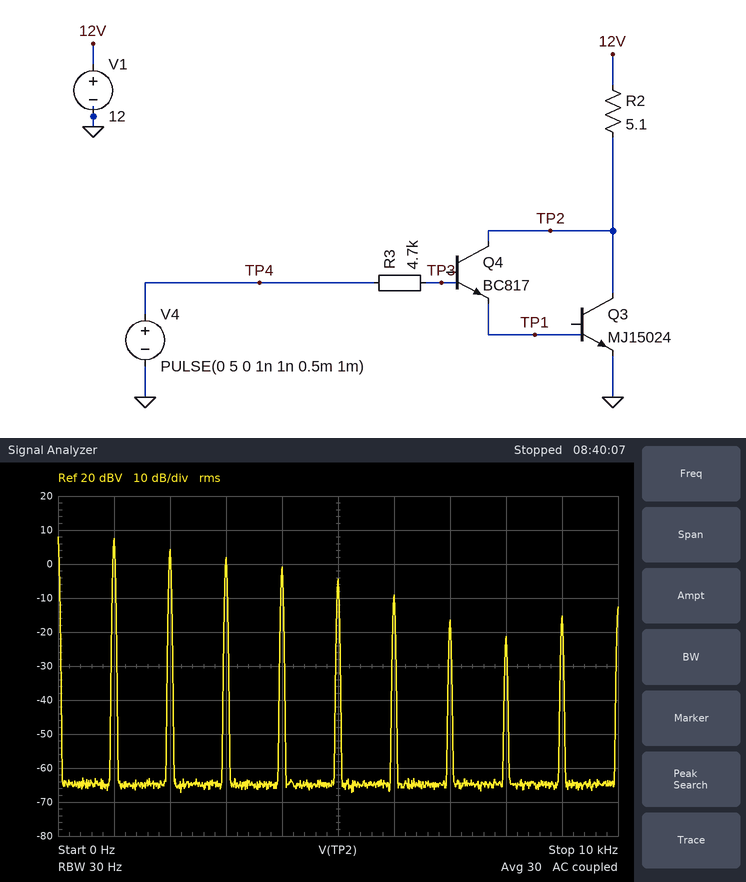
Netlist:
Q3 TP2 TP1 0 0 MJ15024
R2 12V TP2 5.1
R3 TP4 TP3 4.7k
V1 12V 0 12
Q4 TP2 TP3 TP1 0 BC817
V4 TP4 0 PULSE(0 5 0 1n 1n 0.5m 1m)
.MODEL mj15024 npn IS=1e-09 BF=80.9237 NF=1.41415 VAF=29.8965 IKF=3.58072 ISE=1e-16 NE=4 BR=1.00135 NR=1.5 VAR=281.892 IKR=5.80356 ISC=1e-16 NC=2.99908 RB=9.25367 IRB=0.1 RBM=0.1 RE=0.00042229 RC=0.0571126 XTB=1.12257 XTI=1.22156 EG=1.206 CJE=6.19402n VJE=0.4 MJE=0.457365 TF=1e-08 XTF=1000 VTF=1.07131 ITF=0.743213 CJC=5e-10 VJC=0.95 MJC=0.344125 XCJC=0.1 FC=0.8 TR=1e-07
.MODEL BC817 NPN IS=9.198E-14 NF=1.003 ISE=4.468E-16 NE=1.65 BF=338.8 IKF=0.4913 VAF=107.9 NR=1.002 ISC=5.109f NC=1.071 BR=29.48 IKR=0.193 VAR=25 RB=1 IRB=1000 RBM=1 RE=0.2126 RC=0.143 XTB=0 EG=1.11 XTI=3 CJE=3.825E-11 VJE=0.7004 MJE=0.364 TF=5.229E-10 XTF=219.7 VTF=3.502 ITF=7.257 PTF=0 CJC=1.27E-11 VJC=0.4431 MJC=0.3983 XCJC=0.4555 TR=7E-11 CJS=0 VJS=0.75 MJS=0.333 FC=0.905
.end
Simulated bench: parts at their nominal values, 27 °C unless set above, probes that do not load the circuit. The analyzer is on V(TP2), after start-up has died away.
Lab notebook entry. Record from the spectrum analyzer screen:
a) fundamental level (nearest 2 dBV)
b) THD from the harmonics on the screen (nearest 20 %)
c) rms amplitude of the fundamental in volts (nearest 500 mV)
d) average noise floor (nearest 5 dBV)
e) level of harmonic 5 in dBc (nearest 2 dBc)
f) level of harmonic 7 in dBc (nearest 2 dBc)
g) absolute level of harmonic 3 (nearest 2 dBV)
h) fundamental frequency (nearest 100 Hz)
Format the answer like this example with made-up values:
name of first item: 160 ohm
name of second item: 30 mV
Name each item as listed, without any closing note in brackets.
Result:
fundamental level: 8 dBV
THD from the harmonics on the screen: 100 %
rms amplitude of the fundamental in volts: 2.5 V
average noise floor: -65 dBV
level of harmonic 5 in dBc: -12 dBc
level of harmonic 7 in dBc: -24 dBc
absolute level of harmonic 3: 2 dBV
fundamental frequency: 1.0 kHz
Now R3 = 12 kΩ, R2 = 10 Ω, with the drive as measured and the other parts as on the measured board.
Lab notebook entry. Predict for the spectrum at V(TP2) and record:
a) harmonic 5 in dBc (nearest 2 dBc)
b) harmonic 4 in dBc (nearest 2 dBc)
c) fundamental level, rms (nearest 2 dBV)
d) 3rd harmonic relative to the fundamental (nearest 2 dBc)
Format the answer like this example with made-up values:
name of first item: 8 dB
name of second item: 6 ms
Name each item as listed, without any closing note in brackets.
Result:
harmonic 5 in dBc: -24 dBc
harmonic 4 in dBc: -16 dBc
fundamental level, rms: 10 dBV
3rd harmonic relative to the fundamental: -8 dBc
